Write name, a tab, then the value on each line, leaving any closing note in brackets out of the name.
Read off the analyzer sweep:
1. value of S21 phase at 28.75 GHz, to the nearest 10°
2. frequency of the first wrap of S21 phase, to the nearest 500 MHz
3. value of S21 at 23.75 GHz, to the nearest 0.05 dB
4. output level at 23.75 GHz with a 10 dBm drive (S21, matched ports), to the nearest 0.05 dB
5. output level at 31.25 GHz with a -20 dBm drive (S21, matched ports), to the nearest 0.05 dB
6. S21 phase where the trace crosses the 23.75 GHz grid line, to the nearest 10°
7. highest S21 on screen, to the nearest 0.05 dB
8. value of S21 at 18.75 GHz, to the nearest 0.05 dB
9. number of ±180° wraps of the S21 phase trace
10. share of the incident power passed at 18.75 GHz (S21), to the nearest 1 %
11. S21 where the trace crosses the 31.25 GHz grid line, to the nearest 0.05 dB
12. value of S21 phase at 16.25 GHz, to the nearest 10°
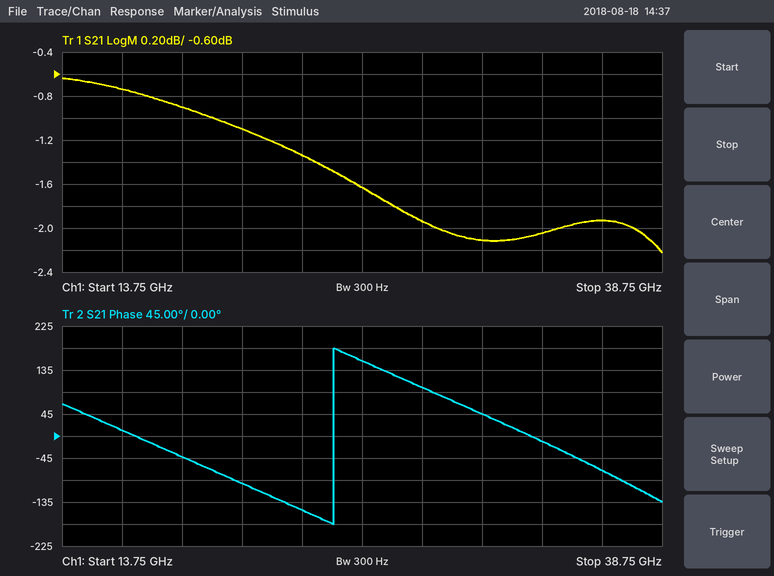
value of S21 phase at 28.75 GHz, to the nearest 10°	100°
frequency of the first wrap of S21 phase, to the nearest 500 MHz	25.0 GHz
value of S21 at 23.75 GHz, to the nearest 0.05 dB	-1.35 dB
output level at 23.75 GHz with a 10 dBm drive (S21, matched ports), to the nearest 0.05 dB	8.65 dBm
output level at 31.25 GHz with a -20 dBm drive (S21, matched ports), to the nearest 0.05 dB	-22.10 dBm
S21 phase where the trace crosses the 23.75 GHz grid line, to the nearest 10°	-150°
highest S21 on screen, to the nearest 0.05 dB	-0.65 dB
value of S21 at 18.75 GHz, to the nearest 0.05 dB	-0.90 dB
number of ±180° wraps of the S21 phase trace	1
share of the incident power passed at 18.75 GHz (S21), to the nearest 1 %	81 %
S21 where the trace crosses the 31.25 GHz grid line, to the nearest 0.05 dB	-2.10 dB
value of S21 phase at 16.25 GHz, to the nearest 10°	10°
